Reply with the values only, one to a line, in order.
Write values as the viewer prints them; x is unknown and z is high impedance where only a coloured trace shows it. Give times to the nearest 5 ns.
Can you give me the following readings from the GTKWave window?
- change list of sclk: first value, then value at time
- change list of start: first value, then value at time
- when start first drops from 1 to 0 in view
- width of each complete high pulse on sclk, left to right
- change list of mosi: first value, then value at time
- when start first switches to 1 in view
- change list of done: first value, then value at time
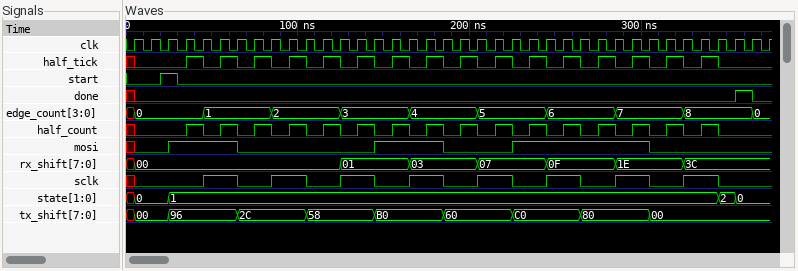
x, 0 at 5 ns, 1 at 45 ns, 0 at 65 ns, 1 at 85 ns, 0 at 105 ns, 1 at 125 ns, 0 at 145 ns, 1 at 165 ns, 0 at 185 ns, 1 at 205 ns, 0 at 225 ns, 1 at 245 ns, 0 at 265 ns, 1 at 285 ns, 0 at 305 ns, 1 at 325 ns, 0 at 345 ns
0, 1 at 20 ns, 0 at 30 ns
30 ns
20 ns, 20 ns, 20 ns, 20 ns, 20 ns, 20 ns, 20 ns, 20 ns
x, 0 at 5 ns, 1 at 25 ns, 0 at 65 ns, 1 at 145 ns, 0 at 185 ns, 1 at 225 ns, 0 at 305 ns
20 ns
x, 0 at 5 ns, 1 at 355 ns, 0 at 365 ns
